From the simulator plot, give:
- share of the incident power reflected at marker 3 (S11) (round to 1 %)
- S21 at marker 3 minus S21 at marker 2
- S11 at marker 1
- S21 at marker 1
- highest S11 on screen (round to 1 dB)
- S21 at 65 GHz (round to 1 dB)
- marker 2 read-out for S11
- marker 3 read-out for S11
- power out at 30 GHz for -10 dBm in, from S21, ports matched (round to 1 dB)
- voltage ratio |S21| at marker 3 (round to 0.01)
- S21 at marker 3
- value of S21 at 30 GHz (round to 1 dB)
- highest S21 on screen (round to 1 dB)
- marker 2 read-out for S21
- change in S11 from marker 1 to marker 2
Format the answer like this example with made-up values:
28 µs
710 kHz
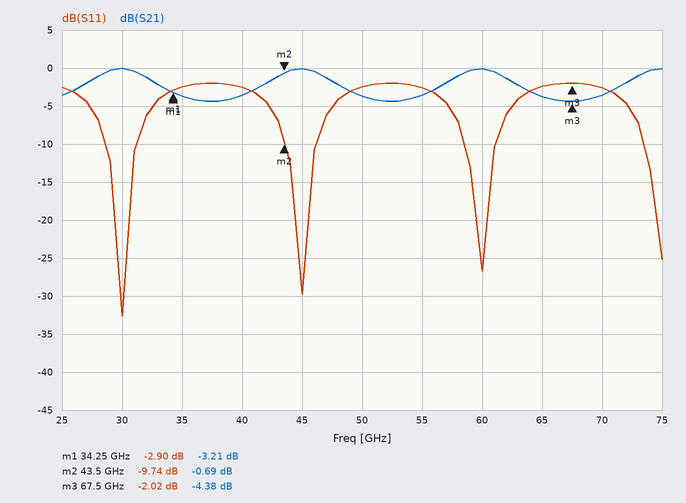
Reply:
63 %
-3.69 dB
-2.90 dB
-3.21 dB
-2 dB
-4 dB
-9.74 dB
-2.02 dB
-10 dBm
0.60
-4.38 dB
0 dB
0 dB
-0.69 dB
-6.84 dB
